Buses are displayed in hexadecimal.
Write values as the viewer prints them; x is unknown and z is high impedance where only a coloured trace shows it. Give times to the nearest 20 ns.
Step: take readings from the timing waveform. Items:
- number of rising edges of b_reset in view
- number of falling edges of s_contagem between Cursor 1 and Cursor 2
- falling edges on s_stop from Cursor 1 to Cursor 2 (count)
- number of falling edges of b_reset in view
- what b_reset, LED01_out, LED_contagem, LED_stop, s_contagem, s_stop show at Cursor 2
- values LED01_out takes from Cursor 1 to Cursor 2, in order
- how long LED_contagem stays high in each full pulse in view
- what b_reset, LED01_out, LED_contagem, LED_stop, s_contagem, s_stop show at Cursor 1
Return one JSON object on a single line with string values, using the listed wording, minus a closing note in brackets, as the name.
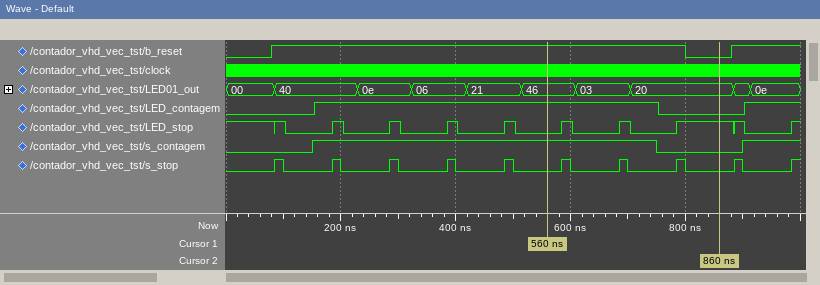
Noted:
{"number of rising edges of b_reset in view": "2", "number of falling edges of s_contagem between Cursor 1 and Cursor 2": "1", "falling edges on s_stop from Cursor 1 to Cursor 2": "3", "number of falling edges of b_reset in view": "1", "what b_reset, LED01_out, LED_contagem, LED_stop, s_contagem, s_stop show at Cursor 2": "b_reset=0, LED01_out=20, LED_contagem=0, LED_stop=1, s_contagem=0, s_stop=0", "values LED01_out takes from Cursor 1 to Cursor 2, in order": "46, 03, 20", "how long LED_contagem stays high in each full pulse in view": "600 ns", "what b_reset, LED01_out, LED_contagem, LED_stop, s_contagem, s_stop show at Cursor 1": "b_reset=1, LED01_out=46, LED_contagem=1, LED_stop=0, s_contagem=1, s_stop=0"}
